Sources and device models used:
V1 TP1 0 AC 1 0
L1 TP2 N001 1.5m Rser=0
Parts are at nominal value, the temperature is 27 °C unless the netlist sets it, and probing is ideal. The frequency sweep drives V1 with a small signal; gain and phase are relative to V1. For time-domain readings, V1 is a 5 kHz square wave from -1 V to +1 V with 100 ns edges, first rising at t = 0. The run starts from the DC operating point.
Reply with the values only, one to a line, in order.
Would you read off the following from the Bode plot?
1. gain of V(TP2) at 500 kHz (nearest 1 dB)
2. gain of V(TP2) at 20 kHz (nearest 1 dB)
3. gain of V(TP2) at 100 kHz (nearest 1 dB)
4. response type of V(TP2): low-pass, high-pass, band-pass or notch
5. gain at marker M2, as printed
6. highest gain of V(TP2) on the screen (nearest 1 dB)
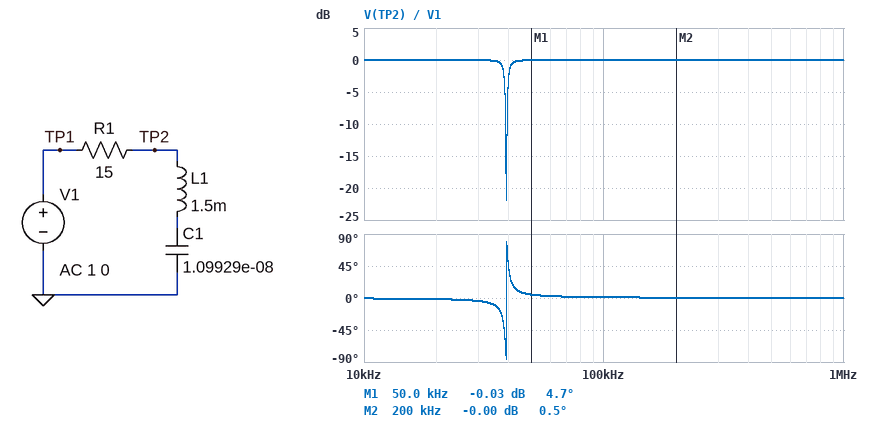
0 dB
0 dB
0 dB
notch
-0.00 dB
0 dB
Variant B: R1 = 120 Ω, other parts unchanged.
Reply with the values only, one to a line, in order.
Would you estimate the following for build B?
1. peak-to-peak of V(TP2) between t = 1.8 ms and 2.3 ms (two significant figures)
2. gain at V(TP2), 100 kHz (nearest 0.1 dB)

2.6 V
-0.1 dB
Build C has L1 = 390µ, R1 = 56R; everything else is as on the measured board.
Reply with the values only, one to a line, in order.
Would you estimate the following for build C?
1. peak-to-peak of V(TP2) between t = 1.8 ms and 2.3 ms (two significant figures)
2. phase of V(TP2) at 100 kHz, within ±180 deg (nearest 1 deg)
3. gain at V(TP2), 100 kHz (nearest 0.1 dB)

2.6 V
29 deg
-1.2 dB
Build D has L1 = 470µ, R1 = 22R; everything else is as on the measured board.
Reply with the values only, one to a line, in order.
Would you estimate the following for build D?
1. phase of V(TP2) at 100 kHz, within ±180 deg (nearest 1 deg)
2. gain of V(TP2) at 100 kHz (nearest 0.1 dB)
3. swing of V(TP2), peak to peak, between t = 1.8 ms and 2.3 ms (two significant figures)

8 deg
-0.1 dB
2.3 V
